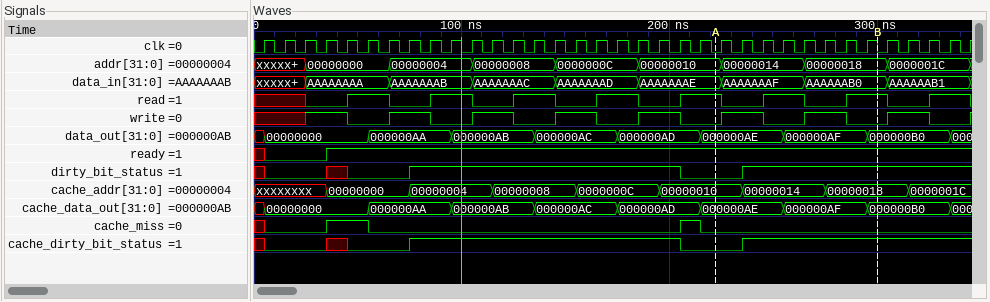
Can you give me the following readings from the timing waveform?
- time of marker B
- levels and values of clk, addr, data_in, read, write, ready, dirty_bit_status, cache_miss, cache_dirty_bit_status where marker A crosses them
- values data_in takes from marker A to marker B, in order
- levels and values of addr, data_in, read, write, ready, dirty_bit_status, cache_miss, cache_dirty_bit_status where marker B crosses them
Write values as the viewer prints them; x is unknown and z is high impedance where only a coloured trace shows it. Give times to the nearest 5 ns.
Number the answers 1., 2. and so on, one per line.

1. 300 ns
2. clk=0, addr=00000010, data_in=AAAAAAAE, read=1, write=0, ready=1, dirty_bit_status=0, cache_miss=0, cache_dirty_bit_status=0
3. AAAAAAAE, AAAAAAAF, AAAAAAB0
4. addr=00000018, data_in=AAAAAAB0, read=1, write=0, ready=1, dirty_bit_status=1, cache_miss=0, cache_dirty_bit_status=1
